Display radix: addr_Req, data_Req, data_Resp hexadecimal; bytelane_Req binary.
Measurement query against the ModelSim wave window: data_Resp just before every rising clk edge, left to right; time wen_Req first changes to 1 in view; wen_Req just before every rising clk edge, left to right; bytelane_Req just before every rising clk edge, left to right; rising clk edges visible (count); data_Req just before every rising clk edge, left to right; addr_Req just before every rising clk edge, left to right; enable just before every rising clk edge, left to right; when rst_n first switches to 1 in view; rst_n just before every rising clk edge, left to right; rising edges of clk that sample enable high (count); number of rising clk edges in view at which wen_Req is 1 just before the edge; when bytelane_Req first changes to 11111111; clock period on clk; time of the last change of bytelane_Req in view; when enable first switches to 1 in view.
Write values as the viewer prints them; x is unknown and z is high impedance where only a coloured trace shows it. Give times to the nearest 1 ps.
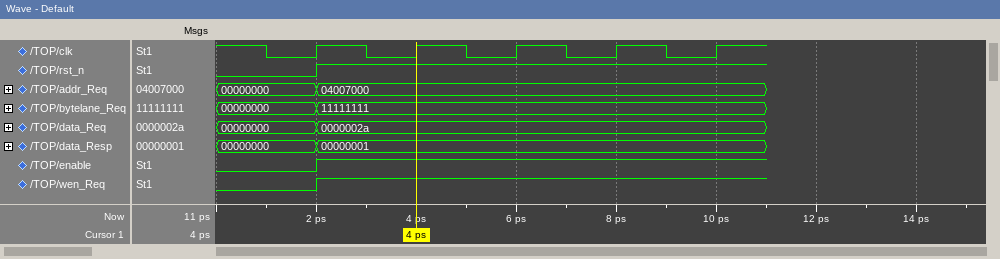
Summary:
00000000, 00000001, 00000001, 00000001, 00000001
2 ps
0 1 1 1 1
00000000, 11111111, 11111111, 11111111, 11111111
5
00000000, 0000002a, 0000002a, 0000002a, 0000002a
00000000, 04007000, 04007000, 04007000, 04007000
0 1 1 1 1
2 ps
0 1 1 1 1
4
4
2 ps
2 ps
2 ps
2 ps
